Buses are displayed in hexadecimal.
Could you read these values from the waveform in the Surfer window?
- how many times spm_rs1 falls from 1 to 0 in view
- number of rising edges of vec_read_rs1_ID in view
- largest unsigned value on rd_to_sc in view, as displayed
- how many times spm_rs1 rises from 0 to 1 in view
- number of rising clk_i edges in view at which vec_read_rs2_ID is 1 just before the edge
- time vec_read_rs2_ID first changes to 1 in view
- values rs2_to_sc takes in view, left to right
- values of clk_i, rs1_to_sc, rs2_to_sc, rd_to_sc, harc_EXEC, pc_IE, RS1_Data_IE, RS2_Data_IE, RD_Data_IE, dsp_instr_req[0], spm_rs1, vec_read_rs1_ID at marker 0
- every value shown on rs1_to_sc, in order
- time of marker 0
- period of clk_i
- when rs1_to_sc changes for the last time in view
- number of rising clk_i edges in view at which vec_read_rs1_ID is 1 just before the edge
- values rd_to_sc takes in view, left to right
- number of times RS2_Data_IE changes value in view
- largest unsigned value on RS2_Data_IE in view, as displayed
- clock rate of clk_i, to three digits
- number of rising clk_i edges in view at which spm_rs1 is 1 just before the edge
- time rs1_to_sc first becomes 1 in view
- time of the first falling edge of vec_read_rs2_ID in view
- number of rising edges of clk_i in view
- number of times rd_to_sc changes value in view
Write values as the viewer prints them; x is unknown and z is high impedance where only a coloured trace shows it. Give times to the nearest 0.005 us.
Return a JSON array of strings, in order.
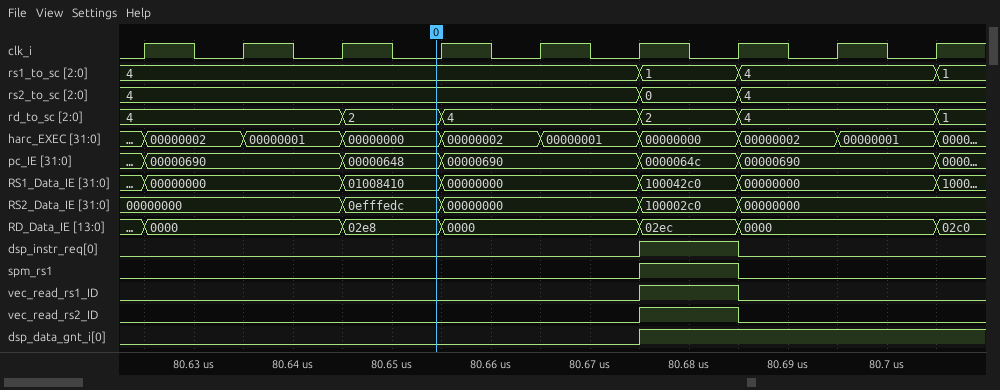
["1", "1", "4", "1", "1", "80.675 us", "4, 0, 4", "clk_i=0, rs1_to_sc=4, rs2_to_sc=4, rd_to_sc=2, harc_EXEC=00000000, pc_IE=00000648, RS1_Data_IE=01008410, RS2_Data_IE=0efffedc, RD_Data_IE=02e8, dsp_instr_req[0]=0, spm_rs1=0, vec_read_rs1_ID=0", "4, 1, 4, 1", "80.655 us", "0.01 us", "80.705 us", "1", "4, 2, 4, 2, 4, 1", "4", "100002c0", "100 MHz", "1", "80.675 us", "80.685 us", "9", "5"]
